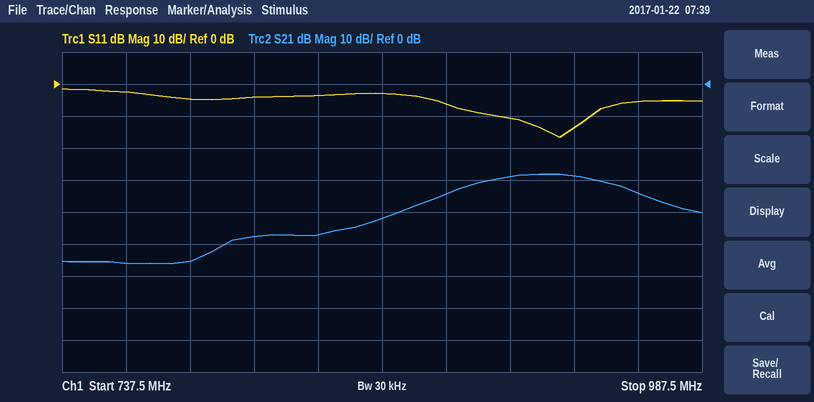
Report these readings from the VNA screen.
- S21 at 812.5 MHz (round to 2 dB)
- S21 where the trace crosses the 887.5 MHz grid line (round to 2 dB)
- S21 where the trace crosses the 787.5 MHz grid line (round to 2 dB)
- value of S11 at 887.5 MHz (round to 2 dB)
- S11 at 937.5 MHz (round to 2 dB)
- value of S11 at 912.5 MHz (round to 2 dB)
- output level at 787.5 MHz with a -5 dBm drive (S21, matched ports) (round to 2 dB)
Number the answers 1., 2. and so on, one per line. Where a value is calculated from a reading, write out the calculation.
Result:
1. -48 dB
2. -34 dB
3. -56 dB
4. -6 dB
5. -14 dB
6. -10 dB
7. -5 dBm + (-56 dB) = -60 dBm
